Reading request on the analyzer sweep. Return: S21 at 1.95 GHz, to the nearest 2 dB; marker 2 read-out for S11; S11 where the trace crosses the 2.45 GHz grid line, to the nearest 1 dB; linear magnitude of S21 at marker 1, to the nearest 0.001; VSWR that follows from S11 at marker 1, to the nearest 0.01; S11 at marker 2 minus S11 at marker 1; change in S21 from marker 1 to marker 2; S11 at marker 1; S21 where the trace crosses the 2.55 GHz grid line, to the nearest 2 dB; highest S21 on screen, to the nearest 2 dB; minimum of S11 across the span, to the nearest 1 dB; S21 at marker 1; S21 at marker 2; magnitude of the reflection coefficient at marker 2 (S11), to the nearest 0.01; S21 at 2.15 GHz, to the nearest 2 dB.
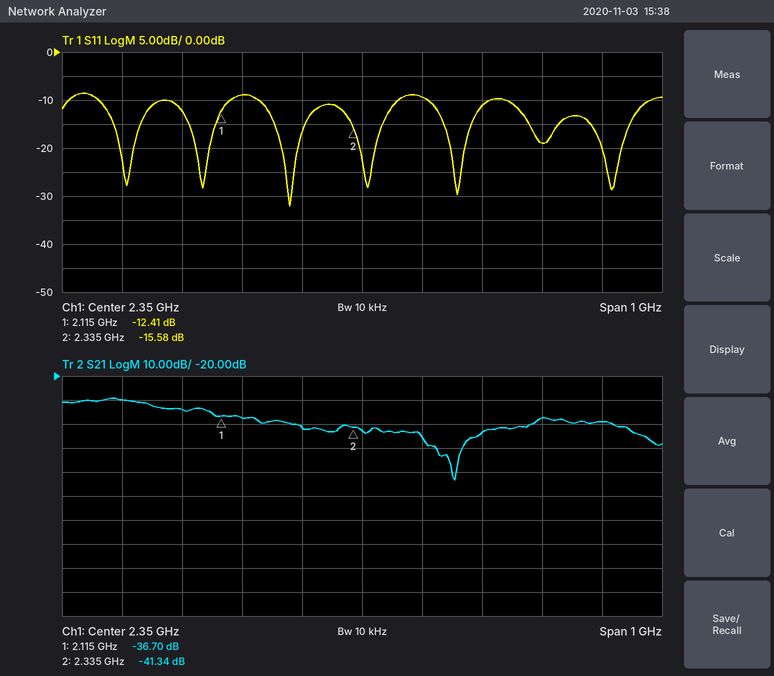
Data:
-30 dB
-15.58 dB
-9 dB
0.015
1.63
-3.17 dB
-4.64 dB
-12.41 dB
-44 dB
-30 dB
-32 dB
-36.70 dB
-41.34 dB
0.17
-38 dB
